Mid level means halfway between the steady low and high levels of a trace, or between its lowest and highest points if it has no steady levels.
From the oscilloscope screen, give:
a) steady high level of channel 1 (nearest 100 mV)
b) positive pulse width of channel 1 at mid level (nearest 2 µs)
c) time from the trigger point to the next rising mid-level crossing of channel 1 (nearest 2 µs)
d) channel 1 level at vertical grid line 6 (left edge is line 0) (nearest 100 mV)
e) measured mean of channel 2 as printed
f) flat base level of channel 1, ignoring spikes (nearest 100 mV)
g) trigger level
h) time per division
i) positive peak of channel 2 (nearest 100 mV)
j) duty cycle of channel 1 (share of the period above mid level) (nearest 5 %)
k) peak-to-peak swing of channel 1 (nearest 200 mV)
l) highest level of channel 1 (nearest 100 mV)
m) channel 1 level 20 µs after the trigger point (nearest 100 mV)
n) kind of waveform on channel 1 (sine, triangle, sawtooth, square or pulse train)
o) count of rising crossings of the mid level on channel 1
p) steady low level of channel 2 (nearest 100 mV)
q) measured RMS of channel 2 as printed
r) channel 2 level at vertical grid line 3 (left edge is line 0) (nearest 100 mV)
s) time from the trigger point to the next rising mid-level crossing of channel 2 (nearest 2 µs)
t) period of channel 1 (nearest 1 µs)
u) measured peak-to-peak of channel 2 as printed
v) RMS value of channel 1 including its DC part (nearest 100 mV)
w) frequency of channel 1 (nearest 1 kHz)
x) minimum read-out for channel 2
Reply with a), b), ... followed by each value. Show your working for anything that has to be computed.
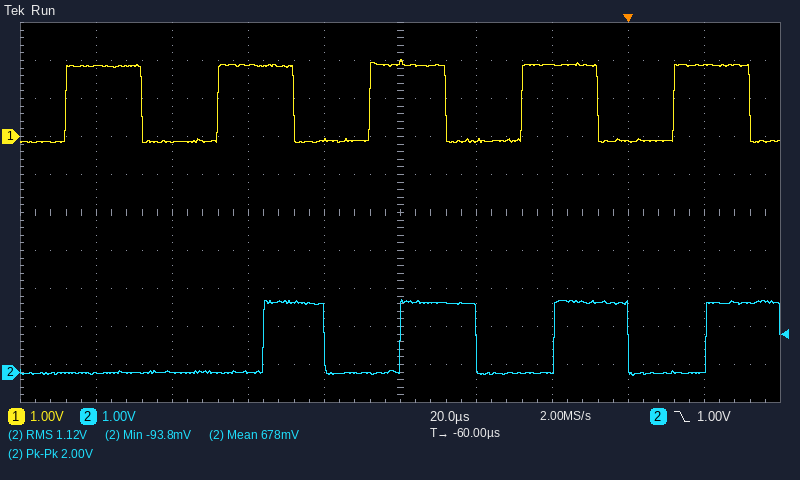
a) 1.9 V
b) 20 µs
c) 12 µs
d) -100 mV
e) 678 mV
f) -100 mV
g) 1.00 V
h) 20 µs
i) 1.9 V
j) 20 µs / 40 µs ≈ 50 %
k) 2.2 V
l) 2.0 V
m) 1.9 V
n) square
o) 5
p) 0.0 V
q) 1.12 V
r) 0.0 V
s) 20 µs
t) 40 µs
u) 2.00 V
v) √(0.5 × (1.9 V)² + 0.5 × (-100 mV)²) ≈ 1.3 V
w) 1 / 40 µs ≈ 25 kHz
x) -93.8 mV
